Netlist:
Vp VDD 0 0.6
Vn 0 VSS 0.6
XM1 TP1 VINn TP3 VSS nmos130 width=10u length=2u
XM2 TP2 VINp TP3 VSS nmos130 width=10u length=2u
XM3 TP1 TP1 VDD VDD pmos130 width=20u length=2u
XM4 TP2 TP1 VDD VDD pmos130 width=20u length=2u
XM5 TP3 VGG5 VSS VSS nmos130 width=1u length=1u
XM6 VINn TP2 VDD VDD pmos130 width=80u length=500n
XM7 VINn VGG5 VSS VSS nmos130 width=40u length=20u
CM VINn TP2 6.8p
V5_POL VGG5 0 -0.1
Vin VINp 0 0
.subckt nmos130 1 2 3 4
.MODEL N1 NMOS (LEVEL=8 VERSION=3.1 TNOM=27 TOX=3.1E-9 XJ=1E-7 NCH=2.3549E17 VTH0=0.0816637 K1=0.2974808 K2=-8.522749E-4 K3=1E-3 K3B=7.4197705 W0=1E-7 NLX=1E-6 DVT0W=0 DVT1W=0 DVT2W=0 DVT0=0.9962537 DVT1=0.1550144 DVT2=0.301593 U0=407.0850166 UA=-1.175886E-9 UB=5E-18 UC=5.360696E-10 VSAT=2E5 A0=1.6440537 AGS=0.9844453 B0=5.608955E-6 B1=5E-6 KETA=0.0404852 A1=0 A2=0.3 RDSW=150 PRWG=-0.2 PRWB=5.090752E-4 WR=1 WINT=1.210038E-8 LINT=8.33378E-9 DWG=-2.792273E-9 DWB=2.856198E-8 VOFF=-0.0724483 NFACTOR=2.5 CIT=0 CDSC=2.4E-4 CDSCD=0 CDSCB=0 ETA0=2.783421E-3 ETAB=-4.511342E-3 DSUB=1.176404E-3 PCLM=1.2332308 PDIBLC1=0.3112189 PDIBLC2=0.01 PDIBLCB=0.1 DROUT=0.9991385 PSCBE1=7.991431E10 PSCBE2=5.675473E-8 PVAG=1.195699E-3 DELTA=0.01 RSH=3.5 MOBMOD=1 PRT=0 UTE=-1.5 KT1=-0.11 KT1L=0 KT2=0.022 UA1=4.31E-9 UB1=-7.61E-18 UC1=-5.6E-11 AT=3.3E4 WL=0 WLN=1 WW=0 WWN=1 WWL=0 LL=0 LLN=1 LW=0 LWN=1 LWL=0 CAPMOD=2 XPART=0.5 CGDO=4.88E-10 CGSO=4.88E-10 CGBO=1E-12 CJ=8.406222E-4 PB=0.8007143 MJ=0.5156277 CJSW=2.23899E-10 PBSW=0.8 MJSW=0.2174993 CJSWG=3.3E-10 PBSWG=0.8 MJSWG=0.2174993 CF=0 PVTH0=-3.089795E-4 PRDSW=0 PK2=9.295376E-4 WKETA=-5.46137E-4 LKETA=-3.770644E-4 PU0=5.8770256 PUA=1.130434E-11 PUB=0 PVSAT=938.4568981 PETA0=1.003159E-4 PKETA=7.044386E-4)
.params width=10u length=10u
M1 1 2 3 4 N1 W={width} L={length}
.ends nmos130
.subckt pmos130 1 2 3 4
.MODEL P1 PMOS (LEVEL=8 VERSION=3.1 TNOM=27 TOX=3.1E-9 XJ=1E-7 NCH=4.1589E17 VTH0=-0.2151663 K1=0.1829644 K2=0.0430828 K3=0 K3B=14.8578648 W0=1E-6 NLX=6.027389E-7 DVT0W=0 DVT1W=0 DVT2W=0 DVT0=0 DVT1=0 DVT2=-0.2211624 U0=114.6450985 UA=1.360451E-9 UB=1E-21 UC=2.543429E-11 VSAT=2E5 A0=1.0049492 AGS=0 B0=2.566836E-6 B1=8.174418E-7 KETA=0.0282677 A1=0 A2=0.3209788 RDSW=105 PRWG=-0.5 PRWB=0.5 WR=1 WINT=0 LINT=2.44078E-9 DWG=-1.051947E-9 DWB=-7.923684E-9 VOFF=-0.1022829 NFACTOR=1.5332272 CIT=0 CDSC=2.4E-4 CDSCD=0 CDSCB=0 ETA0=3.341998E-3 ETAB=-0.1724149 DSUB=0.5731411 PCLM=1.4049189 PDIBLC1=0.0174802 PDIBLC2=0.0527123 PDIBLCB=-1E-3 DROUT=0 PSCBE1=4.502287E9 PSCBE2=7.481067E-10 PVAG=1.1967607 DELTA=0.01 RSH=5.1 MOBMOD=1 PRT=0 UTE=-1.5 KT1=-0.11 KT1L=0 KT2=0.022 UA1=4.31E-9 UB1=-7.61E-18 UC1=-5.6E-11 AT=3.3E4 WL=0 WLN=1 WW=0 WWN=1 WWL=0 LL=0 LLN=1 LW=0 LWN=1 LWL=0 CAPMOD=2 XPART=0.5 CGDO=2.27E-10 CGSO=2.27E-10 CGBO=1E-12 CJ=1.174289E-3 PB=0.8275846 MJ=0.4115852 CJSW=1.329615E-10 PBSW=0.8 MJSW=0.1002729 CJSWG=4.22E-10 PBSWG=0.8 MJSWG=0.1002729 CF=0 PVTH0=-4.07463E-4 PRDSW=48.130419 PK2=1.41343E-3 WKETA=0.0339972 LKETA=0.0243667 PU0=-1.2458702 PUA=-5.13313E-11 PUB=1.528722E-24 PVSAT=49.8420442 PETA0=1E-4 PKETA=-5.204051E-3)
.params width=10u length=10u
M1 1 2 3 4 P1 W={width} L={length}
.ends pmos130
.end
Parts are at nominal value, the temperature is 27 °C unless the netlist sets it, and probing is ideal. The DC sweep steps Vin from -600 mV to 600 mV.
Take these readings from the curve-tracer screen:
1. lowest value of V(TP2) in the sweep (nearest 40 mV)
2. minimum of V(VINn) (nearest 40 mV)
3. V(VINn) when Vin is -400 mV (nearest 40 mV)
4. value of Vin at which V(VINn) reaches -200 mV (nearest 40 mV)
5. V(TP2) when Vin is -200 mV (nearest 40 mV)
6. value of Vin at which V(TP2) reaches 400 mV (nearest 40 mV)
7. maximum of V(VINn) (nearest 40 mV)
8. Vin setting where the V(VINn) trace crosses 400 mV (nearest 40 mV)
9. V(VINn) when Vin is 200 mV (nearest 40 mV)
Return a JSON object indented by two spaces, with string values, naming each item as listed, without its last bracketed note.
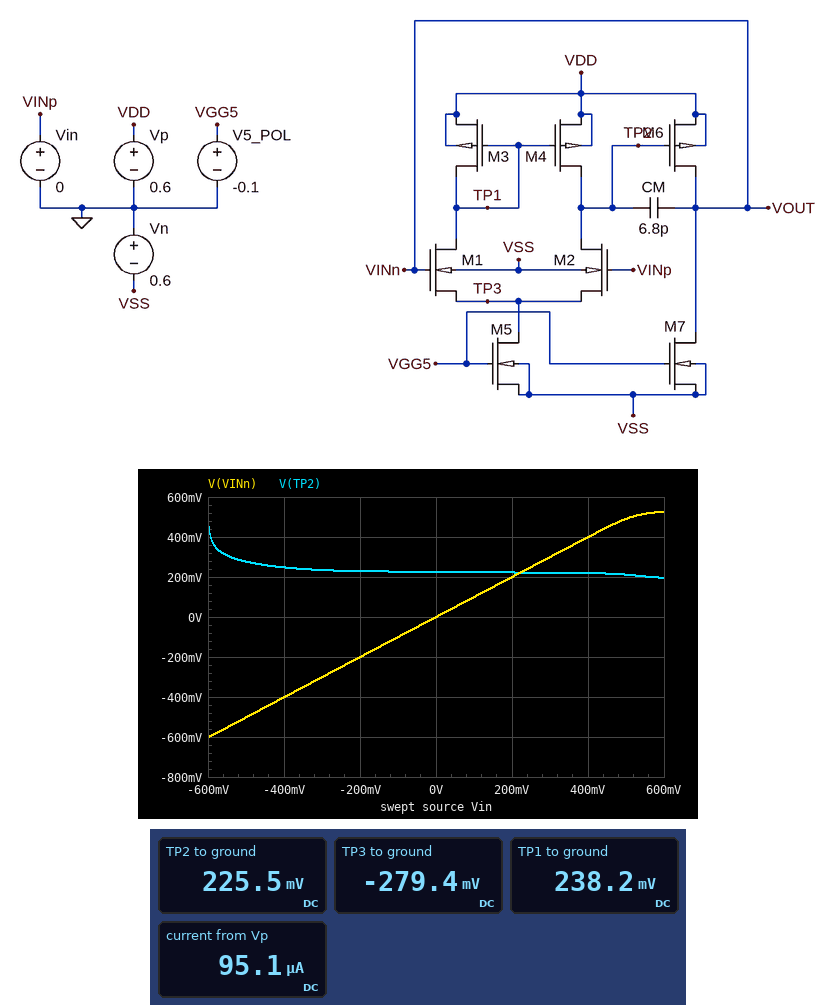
{
  "lowest value of V(TP2) in the sweep": "200 mV",
  "minimum of V(VINn)": "-600 mV",
  "V(VINn) when Vin is -400 mV": "-400 mV",
  "value of Vin at which V(VINn) reaches -200 mV": "-200 mV",
  "V(TP2) when Vin is -200 mV": "240 mV",
  "value of Vin at which V(TP2) reaches 400 mV": "-600 mV",
  "maximum of V(VINn)": "520 mV",
  "Vin setting where the V(VINn) trace crosses 400 mV": "400 mV",
  "V(VINn) when Vin is 200 mV": "200 mV"
}
